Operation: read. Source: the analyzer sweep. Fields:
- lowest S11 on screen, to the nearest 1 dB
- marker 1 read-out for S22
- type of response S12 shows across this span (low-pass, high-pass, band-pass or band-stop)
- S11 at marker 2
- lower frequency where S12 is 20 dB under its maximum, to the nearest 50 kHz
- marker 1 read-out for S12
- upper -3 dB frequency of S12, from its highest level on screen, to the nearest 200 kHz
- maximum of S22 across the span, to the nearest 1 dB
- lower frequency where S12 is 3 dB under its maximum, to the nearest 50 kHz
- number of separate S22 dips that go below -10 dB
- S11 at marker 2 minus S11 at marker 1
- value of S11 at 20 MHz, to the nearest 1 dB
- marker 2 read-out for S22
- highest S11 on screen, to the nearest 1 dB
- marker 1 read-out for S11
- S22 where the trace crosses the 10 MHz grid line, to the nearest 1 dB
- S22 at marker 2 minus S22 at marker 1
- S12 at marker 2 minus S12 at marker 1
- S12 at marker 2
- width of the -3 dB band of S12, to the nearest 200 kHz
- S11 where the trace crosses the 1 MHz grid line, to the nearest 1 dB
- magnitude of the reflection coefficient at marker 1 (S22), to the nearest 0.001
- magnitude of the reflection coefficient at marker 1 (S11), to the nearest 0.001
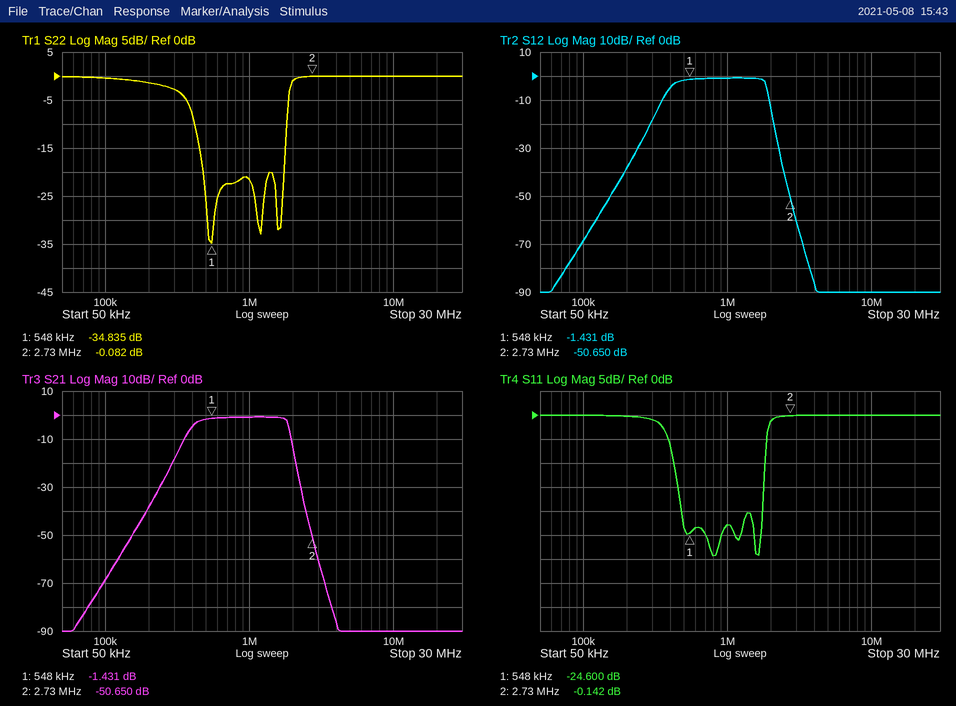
-29 dB
-34.835 dB
band-pass
-0.142 dB
300 kHz
-1.431 dB
1.8 MHz
0 dB
400 kHz
3
24.458 dB
0 dB
-0.082 dB
0 dB
-24.600 dB
0 dB
34.753 dB
-49.219 dB
-50.650 dB
1.4 MHz
-23 dB
0.018
0.059
